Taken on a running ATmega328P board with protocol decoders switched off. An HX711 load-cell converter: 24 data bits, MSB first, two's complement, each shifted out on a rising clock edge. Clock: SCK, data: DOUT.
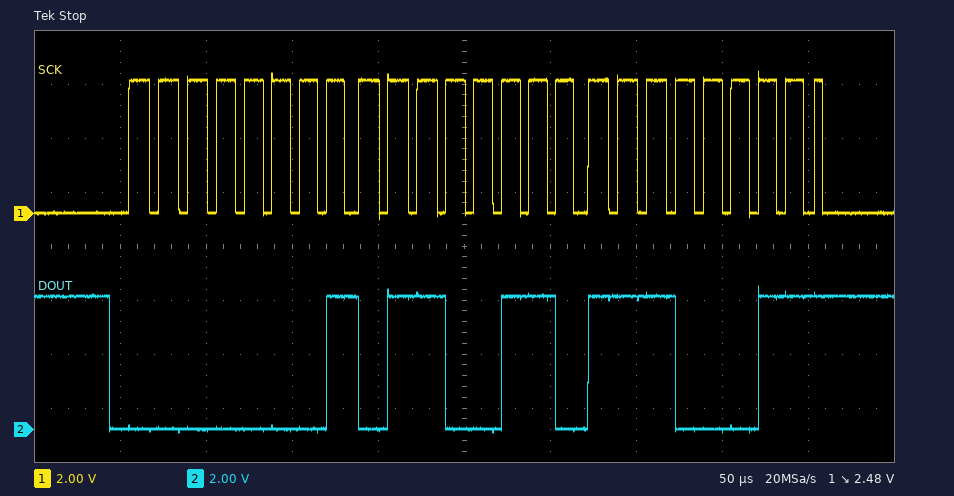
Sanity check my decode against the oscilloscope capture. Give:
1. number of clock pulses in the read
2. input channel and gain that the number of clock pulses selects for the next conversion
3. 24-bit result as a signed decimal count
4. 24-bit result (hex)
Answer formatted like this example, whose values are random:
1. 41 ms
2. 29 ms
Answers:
1. 25
2. channel A, gain 128
3. 91875
4. 0x0166E3
